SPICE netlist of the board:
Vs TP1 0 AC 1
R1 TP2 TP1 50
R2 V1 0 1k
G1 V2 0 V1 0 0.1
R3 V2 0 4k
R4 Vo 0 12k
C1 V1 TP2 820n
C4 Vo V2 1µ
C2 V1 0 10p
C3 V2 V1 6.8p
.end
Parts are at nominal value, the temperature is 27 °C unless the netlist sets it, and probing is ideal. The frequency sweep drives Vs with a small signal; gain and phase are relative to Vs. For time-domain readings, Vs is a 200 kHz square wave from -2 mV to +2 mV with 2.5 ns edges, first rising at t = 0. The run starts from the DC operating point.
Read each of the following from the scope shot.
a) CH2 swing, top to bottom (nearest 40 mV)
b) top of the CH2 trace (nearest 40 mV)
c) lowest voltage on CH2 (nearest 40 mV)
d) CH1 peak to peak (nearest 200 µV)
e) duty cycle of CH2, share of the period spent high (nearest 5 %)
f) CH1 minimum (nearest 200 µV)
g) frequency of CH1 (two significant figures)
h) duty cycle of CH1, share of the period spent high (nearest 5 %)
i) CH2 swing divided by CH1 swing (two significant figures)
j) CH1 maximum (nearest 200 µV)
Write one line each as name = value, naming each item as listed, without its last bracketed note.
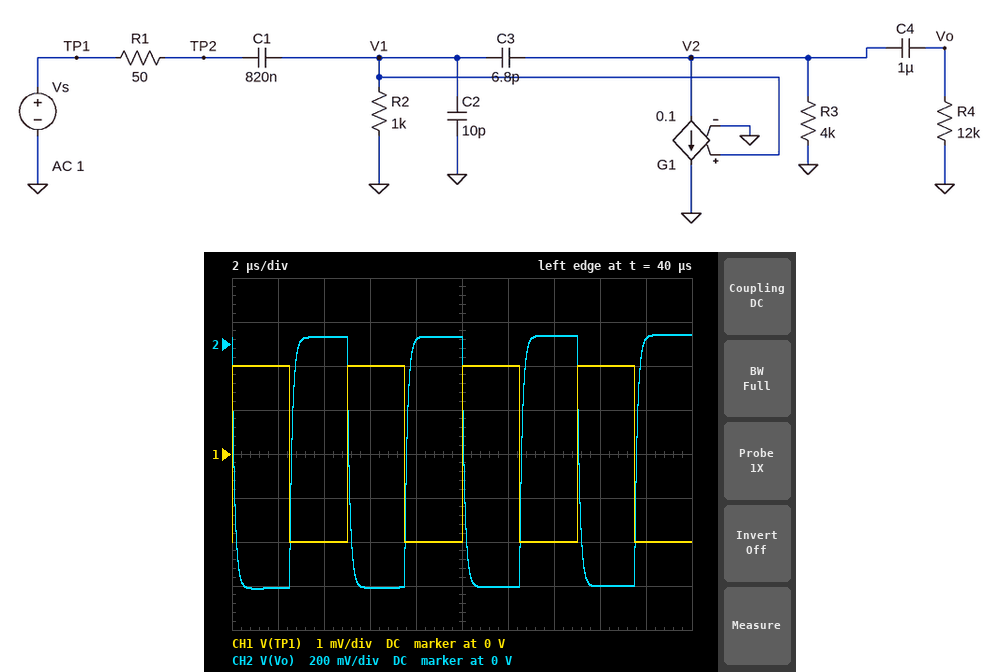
CH2 swing, top to bottom = 1.16 V
top of the CH2 trace = 40 mV
lowest voltage on CH2 = -1.12 V
CH1 peak to peak = 4.0 mV
duty cycle of CH2, share of the period spent high = 50 %
CH1 minimum = -2.0 mV
frequency of CH1 = 200 kHz
duty cycle of CH1, share of the period spent high = 50 %
CH2 swing divided by CH1 swing = 290
CH1 maximum = 2.0 mV
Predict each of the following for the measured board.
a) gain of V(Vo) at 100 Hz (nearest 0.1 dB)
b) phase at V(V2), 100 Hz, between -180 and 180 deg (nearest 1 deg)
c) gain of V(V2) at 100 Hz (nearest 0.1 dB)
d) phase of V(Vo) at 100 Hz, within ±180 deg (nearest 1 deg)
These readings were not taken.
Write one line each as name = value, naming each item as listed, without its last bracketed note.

gain of V(Vo) at 100 Hz = 42.6 dB
phase at V(V2), 100 Hz, between -180 and 180 deg = -120 deg
gain of V(V2) at 100 Hz = 42.7 dB
phase of V(Vo) at 100 Hz, within ±180 deg = -113 deg
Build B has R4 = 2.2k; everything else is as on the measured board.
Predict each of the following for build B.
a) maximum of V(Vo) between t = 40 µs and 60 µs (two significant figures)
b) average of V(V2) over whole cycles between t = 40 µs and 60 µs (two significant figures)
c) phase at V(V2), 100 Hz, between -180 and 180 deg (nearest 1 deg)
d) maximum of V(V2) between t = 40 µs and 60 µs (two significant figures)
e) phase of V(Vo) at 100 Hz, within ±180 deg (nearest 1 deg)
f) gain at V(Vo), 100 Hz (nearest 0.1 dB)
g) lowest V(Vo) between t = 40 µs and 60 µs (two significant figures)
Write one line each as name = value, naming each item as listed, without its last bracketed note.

maximum of V(Vo) between t = 40 µs and 60 µs = 21 mV
average of V(V2) over whole cycles between t = 40 µs and 60 µs = -260 mV
phase at V(V2), 100 Hz, between -180 and 180 deg = -140 deg
maximum of V(V2) between t = 40 µs and 60 µs = 14 mV
phase of V(Vo) at 100 Hz, within ±180 deg = -104 deg
gain at V(Vo), 100 Hz = 35.9 dB
lowest V(Vo) between t = 40 µs and 60 µs = -530 mV
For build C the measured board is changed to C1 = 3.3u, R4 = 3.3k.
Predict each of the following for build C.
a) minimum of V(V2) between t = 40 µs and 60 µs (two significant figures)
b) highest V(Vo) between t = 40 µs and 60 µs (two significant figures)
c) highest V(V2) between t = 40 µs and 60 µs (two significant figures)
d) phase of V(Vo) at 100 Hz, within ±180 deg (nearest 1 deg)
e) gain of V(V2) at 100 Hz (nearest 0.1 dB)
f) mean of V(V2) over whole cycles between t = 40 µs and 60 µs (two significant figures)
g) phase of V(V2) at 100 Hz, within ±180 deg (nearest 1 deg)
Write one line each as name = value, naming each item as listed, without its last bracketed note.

minimum of V(V2) between t = 40 µs and 60 µs = -690 mV
highest V(Vo) between t = 40 µs and 60 µs = 8.7 mV
highest V(V2) between t = 40 µs and 60 µs = 2.5 mV
phase of V(Vo) at 100 Hz, within ±180 deg = -143 deg
gain of V(V2) at 100 Hz = 44.6 dB
mean of V(V2) over whole cycles between t = 40 µs and 60 µs = -340 mV
phase of V(V2) at 100 Hz, within ±180 deg = -169 deg
